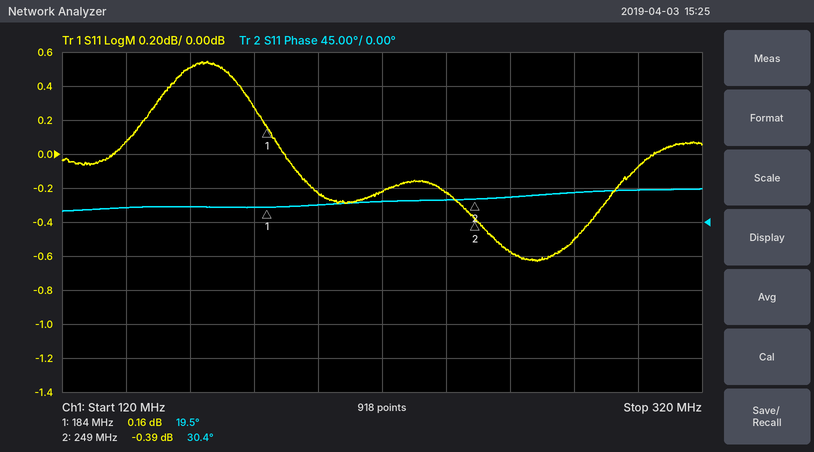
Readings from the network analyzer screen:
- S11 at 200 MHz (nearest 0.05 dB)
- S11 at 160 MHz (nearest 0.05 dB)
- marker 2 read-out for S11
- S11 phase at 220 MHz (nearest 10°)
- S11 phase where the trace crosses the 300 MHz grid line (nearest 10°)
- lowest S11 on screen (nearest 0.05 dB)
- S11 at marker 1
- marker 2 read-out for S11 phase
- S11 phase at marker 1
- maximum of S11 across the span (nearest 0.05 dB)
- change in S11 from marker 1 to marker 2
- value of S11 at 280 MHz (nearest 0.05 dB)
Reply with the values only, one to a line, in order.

-0.25 dB
0.50 dB
-0.39 dB
30°
40°
-0.65 dB
0.16 dB
30.4°
19.5°
0.55 dB
-0.55 dB
-0.50 dB
